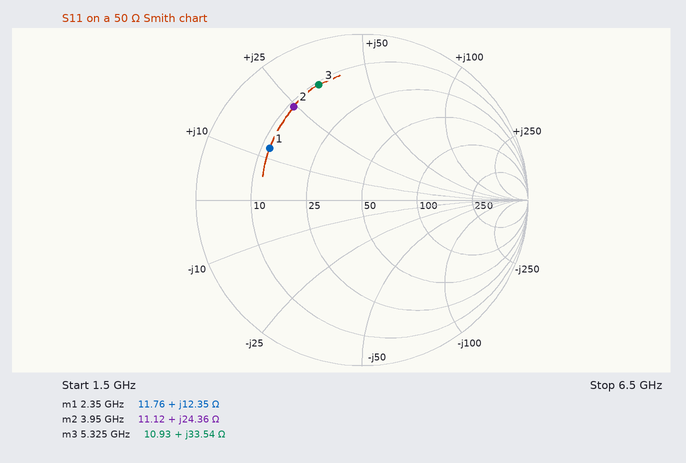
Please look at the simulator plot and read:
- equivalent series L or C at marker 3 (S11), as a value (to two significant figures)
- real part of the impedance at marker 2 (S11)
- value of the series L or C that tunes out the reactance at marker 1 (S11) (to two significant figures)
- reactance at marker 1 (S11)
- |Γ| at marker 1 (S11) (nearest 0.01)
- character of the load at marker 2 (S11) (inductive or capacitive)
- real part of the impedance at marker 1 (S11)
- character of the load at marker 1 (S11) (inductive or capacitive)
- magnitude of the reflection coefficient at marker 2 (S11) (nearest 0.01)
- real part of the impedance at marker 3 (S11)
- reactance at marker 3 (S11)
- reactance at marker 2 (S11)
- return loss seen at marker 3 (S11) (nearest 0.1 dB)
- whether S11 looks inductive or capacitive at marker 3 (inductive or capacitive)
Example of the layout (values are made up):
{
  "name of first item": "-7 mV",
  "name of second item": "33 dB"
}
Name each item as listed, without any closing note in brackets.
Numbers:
{
  "equivalent series L or C at marker 3 (S11), as a value": "1.0 nH",
  "real part of the impedance at marker 2": "11.12 Ω",
  "value of the series L or C that tunes out the reactance at marker 1 (S11)": "5.5 pF",
  "reactance at marker 1": "+12.35 Ω",
  "|Γ| at marker 1 (S11)": "0.64",
  "character of the load at marker 2 (S11)": "inductive",
  "real part of the impedance at marker 1": "11.76 Ω",
  "character of the load at marker 1 (S11)": "inductive",
  "magnitude of the reflection coefficient at marker 2 (S11)": "0.70",
  "real part of the impedance at marker 3": "10.93 Ω",
  "reactance at marker 3": "+33.54 Ω",
  "reactance at marker 2": "+24.36 Ω",
  "return loss seen at marker 3 (S11)": "2.6 dB",
  "whether S11 looks inductive or capacitive at marker 3": "inductive"
}
